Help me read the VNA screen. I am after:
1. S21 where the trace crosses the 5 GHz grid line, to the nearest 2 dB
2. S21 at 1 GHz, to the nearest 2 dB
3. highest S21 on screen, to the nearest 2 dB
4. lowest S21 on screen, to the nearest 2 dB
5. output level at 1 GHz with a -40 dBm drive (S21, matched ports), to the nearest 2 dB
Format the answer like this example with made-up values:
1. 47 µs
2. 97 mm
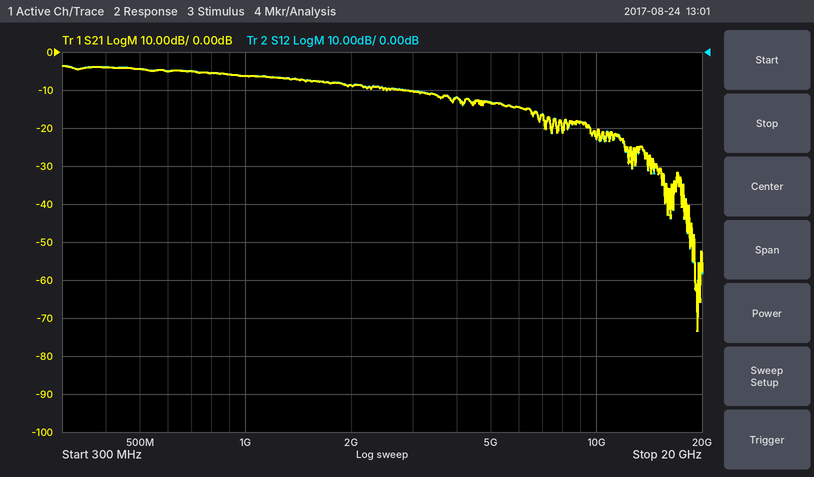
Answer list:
1. -14 dB
2. -6 dB
3. -4 dB
4. -74 dB
5. -46 dBm
